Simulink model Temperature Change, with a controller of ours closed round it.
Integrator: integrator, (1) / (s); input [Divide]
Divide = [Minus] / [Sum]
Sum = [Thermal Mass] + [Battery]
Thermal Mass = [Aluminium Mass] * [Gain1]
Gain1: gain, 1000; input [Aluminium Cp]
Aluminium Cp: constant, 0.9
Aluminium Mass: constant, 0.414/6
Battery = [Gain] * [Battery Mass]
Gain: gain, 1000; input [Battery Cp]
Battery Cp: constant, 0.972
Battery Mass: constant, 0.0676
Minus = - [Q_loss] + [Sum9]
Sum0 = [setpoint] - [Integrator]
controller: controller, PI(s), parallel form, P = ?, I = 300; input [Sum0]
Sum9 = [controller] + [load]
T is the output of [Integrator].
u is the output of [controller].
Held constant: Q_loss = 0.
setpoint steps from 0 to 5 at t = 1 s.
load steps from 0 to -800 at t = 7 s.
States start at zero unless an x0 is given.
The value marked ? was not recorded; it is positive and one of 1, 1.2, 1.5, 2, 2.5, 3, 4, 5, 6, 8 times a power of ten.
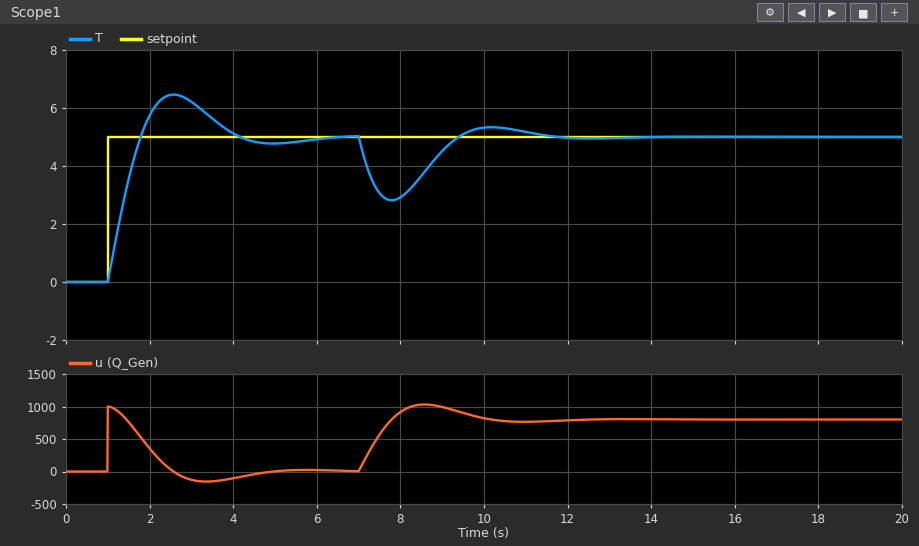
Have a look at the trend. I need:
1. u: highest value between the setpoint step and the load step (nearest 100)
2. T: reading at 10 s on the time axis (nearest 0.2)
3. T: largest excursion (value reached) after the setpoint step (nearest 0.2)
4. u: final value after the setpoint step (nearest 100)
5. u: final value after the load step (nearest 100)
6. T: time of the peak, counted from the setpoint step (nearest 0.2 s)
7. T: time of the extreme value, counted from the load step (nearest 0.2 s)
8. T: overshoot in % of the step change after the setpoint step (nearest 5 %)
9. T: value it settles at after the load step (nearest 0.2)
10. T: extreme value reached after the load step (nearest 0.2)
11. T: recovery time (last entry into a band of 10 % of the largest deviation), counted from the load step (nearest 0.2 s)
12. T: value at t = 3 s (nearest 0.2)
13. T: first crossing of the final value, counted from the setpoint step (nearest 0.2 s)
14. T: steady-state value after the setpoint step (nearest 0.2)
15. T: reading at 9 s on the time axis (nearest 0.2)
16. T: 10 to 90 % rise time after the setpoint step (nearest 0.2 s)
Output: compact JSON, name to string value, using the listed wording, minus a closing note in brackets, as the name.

{"u: highest value between the setpoint step and the load step": "1000", "T: reading at 10 s on the time axis": "5.4", "T: largest excursion (value reached) after the setpoint step": "6.4", "u: final value after the setpoint step": "0", "u: final value after the load step": "800", "T: time of the peak, counted from the setpoint step": "1.6 s", "T: time of the extreme value, counted from the load step": "0.8 s", "T: overshoot in % of the step change after the setpoint step": "30 %", "T: value it settles at after the load step": "5.0", "T: extreme value reached after the load step": "2.8", "T: recovery time (last entry into a band of 10 % of the largest deviation), counted from the load step": "3.8 s", "T: value at t = 3 s": "6.2", "T: first crossing of the final value, counted from the setpoint step": "0.8 s", "T: steady-state value after the setpoint step": "5.0", "T: reading at 9 s on the time axis": "4.6", "T: 10 to 90 % rise time after the setpoint step": "0.6 s"}
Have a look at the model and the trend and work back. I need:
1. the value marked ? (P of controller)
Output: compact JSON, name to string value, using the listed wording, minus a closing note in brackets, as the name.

{"the value marked ?": "200"}
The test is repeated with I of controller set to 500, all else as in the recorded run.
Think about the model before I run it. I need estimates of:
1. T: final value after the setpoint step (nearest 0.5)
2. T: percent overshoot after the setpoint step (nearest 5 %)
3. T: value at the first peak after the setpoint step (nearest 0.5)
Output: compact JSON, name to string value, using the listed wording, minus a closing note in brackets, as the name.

{"T: final value after the setpoint step": "5.0", "T: percent overshoot after the setpoint step": "35 %", "T: value at the first peak after the setpoint step": "7.0"}
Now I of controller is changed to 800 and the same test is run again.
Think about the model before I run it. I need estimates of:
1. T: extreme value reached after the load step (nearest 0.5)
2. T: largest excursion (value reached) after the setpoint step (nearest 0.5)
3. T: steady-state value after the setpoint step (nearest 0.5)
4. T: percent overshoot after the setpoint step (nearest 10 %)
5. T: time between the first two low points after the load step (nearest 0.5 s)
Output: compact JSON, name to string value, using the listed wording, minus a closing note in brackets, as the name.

{"T: extreme value reached after the load step": "3.5", "T: largest excursion (value reached) after the setpoint step": "7.0", "T: steady-state value after the setpoint step": "5.0", "T: percent overshoot after the setpoint step": "40 %", "T: time between the first two low points after the load step": "2.5 s"}
